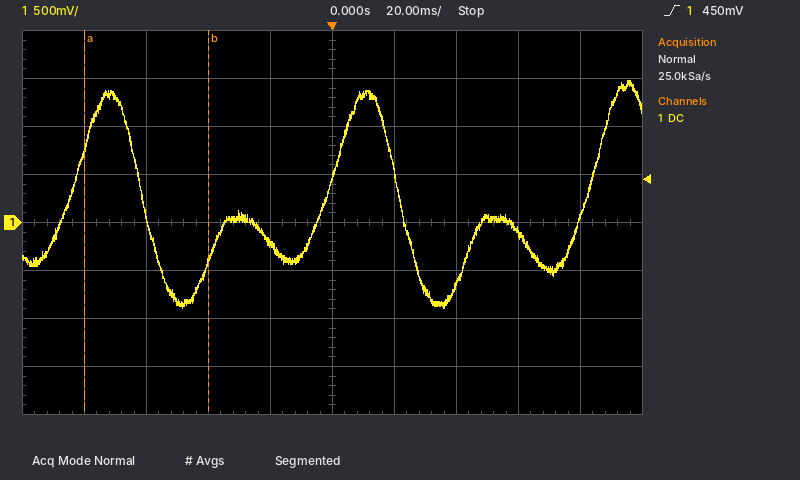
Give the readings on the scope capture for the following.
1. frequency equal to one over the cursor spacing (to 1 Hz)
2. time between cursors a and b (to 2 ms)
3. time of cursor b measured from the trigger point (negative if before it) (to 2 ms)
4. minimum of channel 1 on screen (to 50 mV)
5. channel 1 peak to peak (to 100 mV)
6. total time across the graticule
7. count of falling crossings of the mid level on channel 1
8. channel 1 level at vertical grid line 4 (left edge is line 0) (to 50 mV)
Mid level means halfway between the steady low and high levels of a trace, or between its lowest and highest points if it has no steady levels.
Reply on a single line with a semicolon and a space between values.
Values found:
25 Hz; 40 ms; -40 ms; -900 mV; 2.40 V; 200 ms; 2; -200 mV
